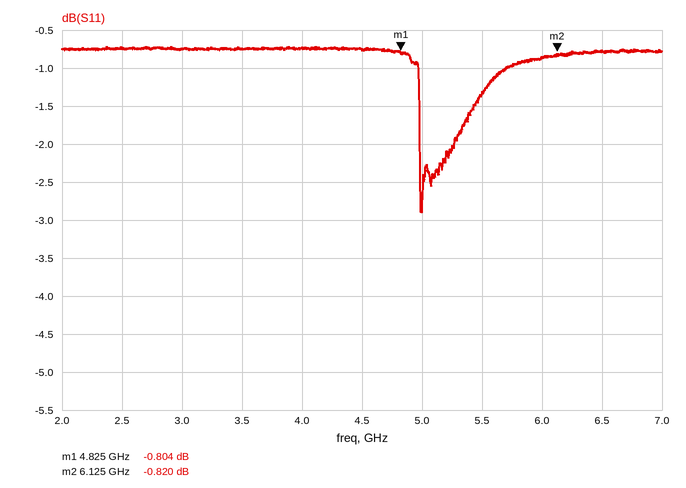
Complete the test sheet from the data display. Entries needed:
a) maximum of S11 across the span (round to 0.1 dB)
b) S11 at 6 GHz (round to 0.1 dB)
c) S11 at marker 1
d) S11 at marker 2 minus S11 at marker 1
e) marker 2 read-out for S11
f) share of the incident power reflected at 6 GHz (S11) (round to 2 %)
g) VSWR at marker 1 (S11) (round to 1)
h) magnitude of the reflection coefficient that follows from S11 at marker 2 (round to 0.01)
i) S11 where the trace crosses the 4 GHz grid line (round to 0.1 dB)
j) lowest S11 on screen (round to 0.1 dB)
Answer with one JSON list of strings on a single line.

["-0.7 dB", "-0.9 dB", "-0.804 dB", "-0.016 dB", "-0.820 dB", "82 %", "22", "0.91", "-0.7 dB", "-2.9 dB"]
